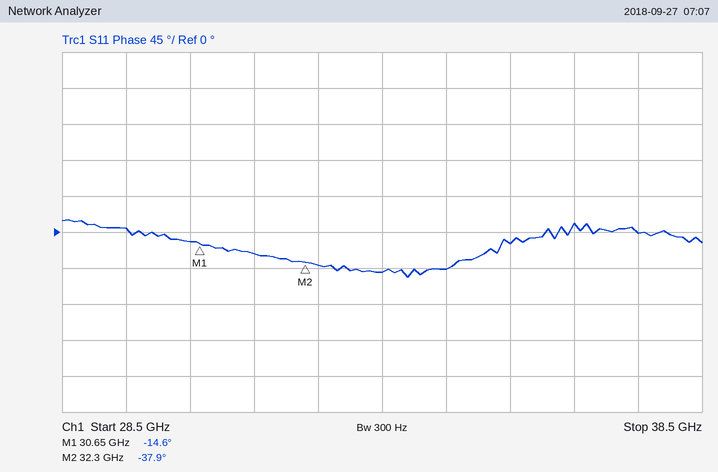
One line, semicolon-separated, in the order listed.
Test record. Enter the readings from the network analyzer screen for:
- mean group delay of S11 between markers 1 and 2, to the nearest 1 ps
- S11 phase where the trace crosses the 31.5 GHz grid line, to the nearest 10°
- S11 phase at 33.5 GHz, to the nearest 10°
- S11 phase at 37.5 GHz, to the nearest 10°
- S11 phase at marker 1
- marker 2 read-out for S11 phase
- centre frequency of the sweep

39 ps; -30°; -50°; 0°; -14.6°; -37.9°; 33.5 GHz
